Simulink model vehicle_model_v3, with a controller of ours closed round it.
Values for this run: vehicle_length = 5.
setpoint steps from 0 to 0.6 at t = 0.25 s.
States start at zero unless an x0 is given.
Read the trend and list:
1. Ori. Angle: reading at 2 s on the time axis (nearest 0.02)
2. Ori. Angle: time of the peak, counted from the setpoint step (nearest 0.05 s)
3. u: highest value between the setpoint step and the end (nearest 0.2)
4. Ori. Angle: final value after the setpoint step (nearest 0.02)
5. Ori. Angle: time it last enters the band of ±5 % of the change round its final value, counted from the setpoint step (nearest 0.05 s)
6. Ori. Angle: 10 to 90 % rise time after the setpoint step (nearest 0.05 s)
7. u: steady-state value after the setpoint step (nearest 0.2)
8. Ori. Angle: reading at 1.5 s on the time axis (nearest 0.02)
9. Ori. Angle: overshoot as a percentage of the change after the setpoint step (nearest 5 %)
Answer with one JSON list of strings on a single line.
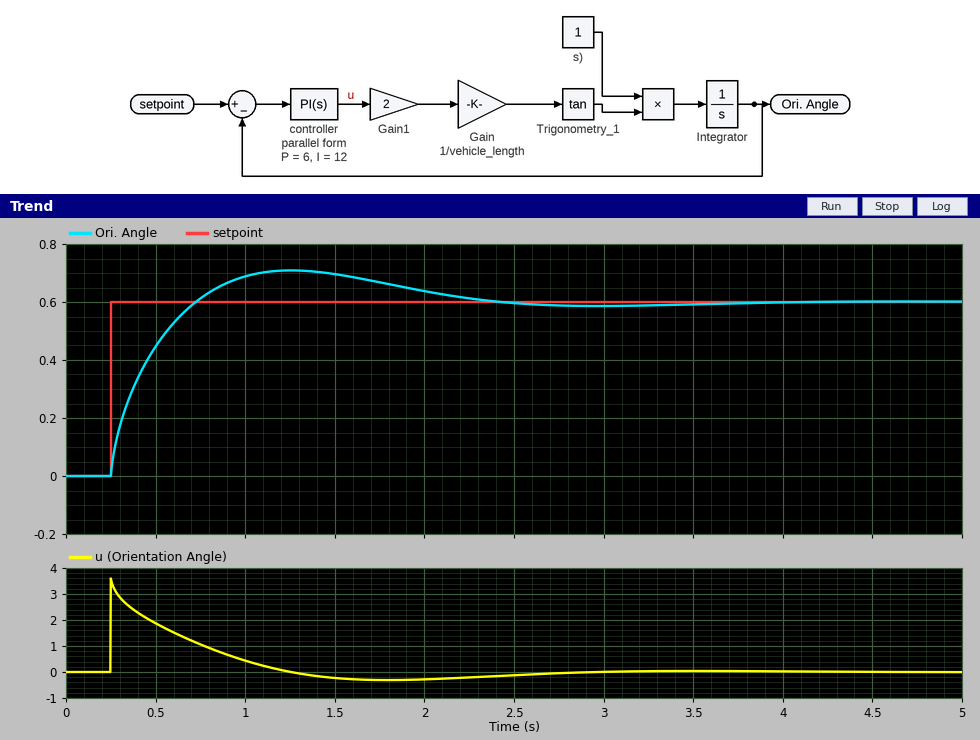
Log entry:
["0.64", "1.00 s", "3.6", "0.60", "1.80 s", "0.35 s", "0.0", "0.70", "20 %"]
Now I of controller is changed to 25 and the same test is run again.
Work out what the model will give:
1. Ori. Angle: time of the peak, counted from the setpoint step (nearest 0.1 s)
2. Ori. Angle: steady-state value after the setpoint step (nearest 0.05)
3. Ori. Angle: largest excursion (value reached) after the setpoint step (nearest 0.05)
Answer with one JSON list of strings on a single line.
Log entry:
["0.7 s", "0.60", "0.75"]
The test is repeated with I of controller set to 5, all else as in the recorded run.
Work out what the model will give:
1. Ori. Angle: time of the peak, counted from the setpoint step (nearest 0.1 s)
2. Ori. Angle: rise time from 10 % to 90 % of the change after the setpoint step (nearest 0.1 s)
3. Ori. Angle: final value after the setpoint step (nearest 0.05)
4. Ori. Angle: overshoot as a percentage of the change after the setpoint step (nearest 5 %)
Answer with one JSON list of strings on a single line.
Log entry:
["1.4 s", "0.5 s", "0.60", "10 %"]
